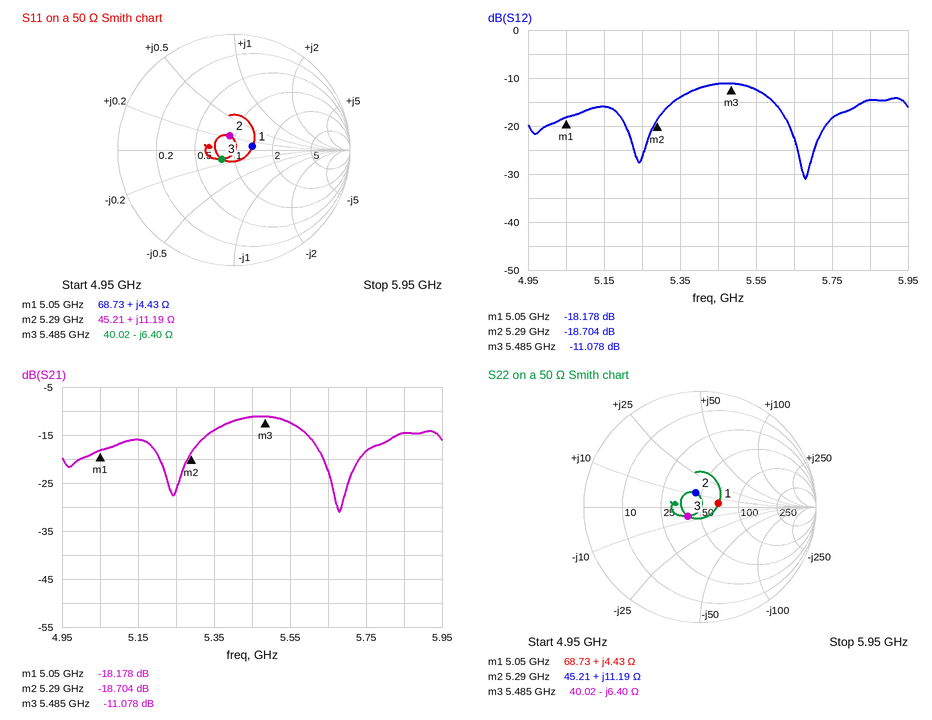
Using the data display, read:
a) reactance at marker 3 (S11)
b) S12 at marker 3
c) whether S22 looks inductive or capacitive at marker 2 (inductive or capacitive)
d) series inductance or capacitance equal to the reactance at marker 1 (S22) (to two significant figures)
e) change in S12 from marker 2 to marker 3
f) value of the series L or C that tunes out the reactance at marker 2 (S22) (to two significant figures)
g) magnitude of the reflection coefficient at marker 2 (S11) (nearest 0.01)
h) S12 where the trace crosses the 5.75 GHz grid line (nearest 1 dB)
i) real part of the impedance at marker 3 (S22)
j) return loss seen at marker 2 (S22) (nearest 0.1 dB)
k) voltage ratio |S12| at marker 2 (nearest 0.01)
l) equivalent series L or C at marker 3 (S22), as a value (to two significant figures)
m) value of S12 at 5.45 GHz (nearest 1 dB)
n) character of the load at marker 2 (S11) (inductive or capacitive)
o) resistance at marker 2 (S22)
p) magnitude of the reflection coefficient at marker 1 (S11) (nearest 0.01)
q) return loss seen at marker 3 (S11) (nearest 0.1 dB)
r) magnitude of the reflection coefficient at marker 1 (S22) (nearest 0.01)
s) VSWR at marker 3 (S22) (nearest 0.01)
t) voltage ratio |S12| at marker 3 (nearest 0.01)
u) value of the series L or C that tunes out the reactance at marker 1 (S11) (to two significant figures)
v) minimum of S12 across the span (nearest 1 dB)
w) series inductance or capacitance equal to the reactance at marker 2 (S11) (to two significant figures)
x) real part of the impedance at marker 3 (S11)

-6.40 Ω
-11.078 dB
inductive
140 pH
7.626 dB
2.7 pF
0.13
-18 dB
40.02 Ω
17.9 dB
0.12
4.5 pF
-11 dB
inductive
45.21 Ω
0.16
17.6 dB
0.16
1.30
0.28
7.1 pF
-31 dB
340 pH
40.02 Ω
